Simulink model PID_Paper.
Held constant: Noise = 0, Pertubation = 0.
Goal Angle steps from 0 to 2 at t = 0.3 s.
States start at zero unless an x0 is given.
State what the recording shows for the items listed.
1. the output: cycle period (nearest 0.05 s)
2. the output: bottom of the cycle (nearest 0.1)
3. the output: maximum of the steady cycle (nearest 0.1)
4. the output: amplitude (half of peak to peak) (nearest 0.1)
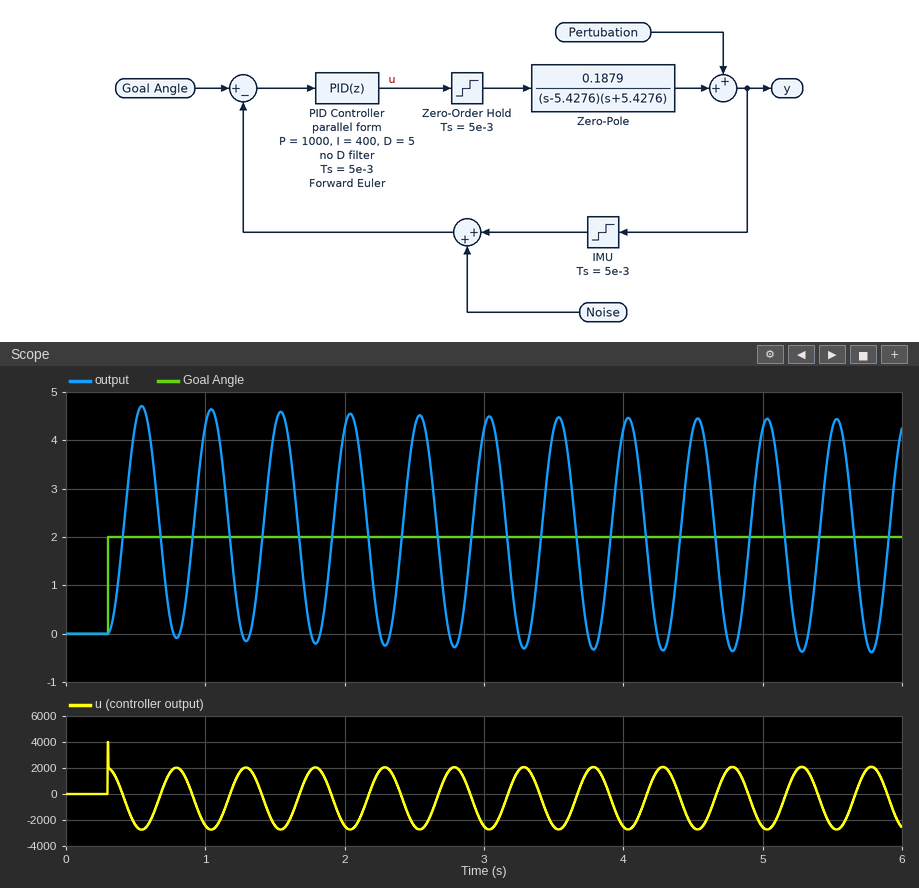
0.50 s
-0.4
4.5
2.4
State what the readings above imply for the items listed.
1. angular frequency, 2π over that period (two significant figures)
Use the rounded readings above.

13 rad/s
